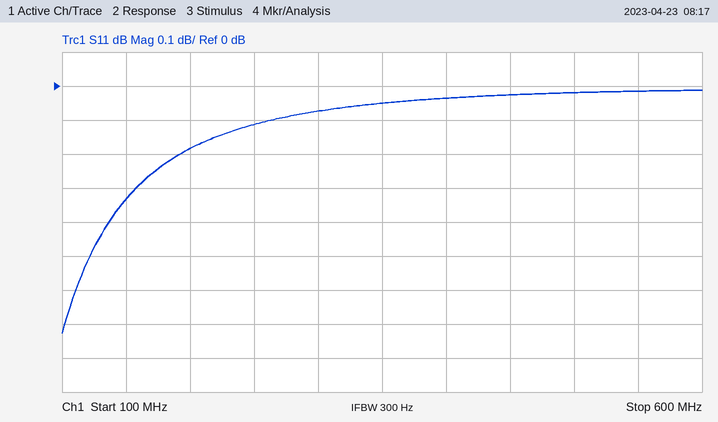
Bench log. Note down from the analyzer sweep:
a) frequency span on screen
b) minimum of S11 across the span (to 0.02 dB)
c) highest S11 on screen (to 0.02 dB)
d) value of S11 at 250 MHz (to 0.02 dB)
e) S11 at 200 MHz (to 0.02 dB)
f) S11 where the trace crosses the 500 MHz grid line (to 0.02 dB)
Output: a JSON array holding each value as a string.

["500 MHz", "-0.72 dB", "-0.02 dB", "-0.12 dB", "-0.18 dB", "-0.02 dB"]
